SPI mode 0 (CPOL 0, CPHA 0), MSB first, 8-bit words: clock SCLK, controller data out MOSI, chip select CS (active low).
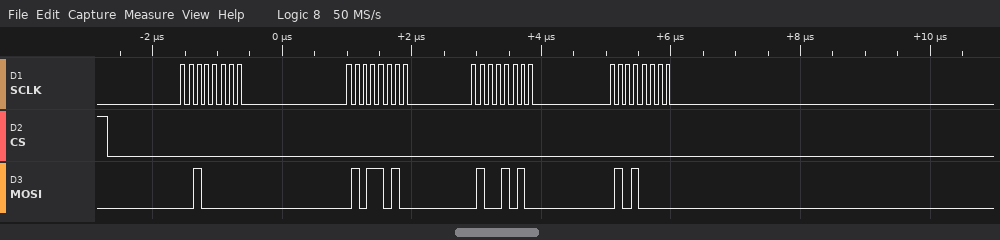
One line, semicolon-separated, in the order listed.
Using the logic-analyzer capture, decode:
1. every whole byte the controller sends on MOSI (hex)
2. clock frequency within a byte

20 5A 4A 50; 8 MHz
